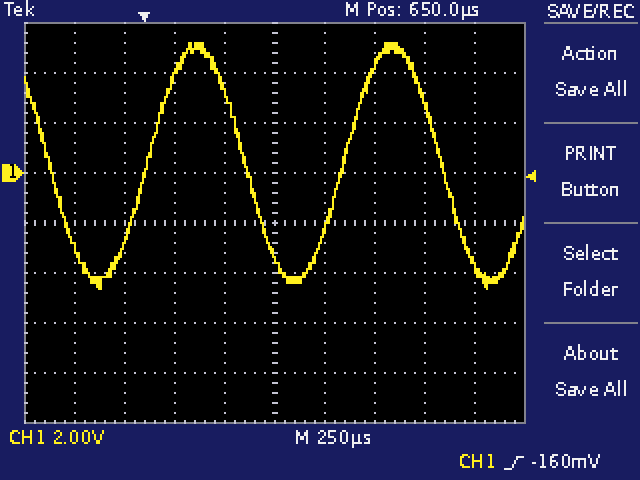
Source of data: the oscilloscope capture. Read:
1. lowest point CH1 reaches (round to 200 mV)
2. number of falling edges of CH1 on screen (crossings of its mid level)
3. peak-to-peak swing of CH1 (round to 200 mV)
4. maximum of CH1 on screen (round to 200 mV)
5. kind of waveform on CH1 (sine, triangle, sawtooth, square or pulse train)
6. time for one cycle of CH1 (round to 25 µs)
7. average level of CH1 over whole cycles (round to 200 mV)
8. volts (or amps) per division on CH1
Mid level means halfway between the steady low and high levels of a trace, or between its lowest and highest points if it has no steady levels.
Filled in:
-4.6 V
3
9.8 V
5.2 V
sine
975 µs
400 mV
2 V
